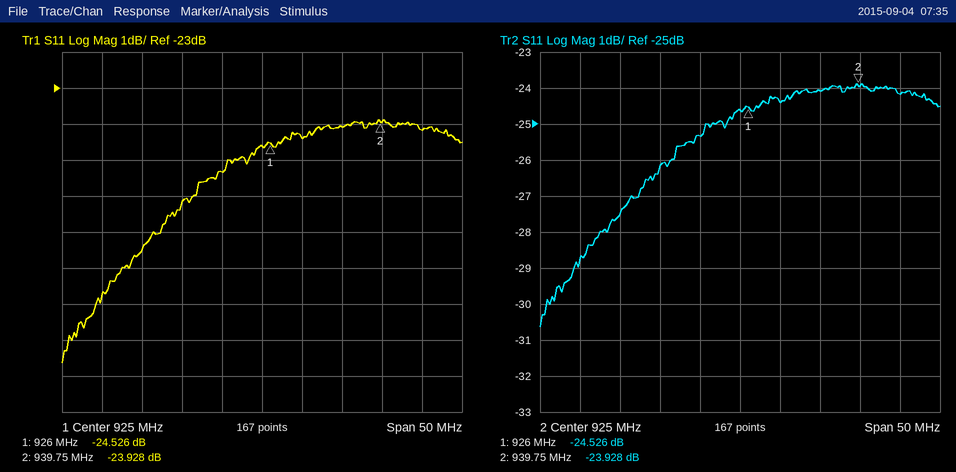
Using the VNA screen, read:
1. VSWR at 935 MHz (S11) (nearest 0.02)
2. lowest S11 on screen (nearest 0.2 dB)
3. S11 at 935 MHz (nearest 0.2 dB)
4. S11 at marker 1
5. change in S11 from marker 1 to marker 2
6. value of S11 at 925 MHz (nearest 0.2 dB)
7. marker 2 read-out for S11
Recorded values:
1.14
-30.6 dB
-24.0 dB
-24.526 dB
0.598 dB
-24.6 dB
-23.928 dB
